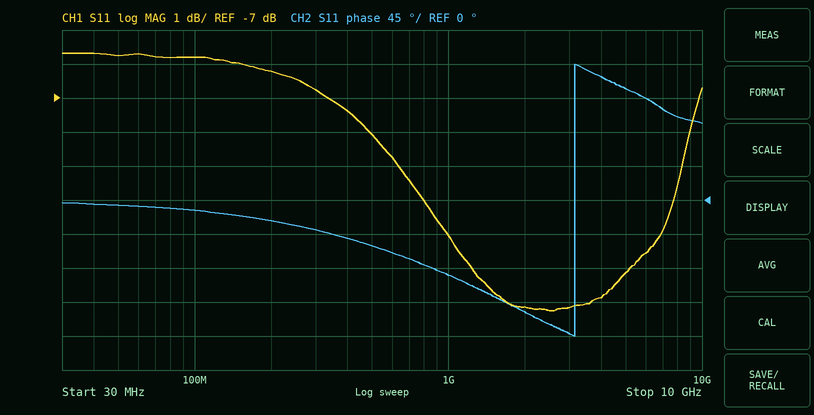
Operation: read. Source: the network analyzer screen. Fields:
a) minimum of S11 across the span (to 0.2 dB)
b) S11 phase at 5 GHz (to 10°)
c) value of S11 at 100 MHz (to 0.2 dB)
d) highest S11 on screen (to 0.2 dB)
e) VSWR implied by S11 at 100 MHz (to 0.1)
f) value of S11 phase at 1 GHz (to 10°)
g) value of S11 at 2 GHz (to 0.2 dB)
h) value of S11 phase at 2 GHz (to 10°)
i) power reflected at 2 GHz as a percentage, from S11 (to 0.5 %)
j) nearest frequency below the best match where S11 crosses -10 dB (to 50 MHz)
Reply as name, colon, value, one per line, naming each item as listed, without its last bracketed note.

minimum of S11 across the span: -13.2 dB
S11 phase at 5 GHz: 150°
value of S11 at 100 MHz: -5.8 dB
highest S11 on screen: -5.6 dB
VSWR implied by S11 at 100 MHz: 3.1
value of S11 phase at 1 GHz: -100°
value of S11 at 2 GHz: -13.2 dB
value of S11 phase at 2 GHz: -150°
power reflected at 2 GHz as a percentage, from S11: 5.0 %
nearest frequency below the best match where S11 crosses -10 dB: 800 MHz
